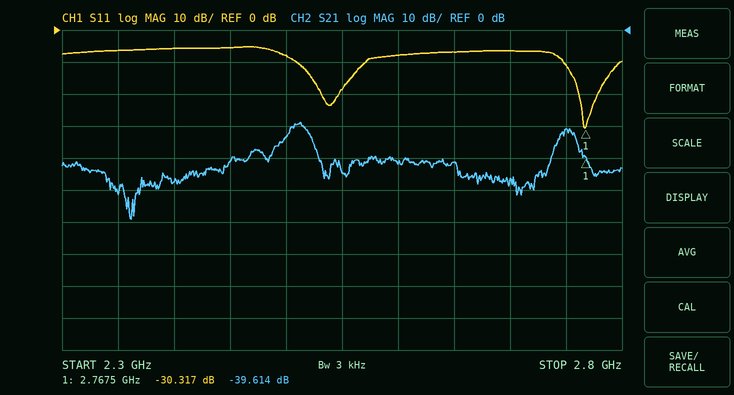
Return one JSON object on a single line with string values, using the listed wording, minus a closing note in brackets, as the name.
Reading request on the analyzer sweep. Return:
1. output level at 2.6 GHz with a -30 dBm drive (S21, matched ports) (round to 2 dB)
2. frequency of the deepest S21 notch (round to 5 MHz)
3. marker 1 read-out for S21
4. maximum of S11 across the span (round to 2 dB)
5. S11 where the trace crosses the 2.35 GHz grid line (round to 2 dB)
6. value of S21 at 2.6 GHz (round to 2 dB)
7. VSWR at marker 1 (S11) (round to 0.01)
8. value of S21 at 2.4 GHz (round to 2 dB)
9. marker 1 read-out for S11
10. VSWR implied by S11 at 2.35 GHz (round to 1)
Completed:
{"output level at 2.6 GHz with a -30 dBm drive (S21, matched ports)": "-72 dBm", "frequency of the deepest S21 notch": "2.360 GHz", "marker 1 read-out for S21": "-39.614 dB", "maximum of S11 across the span": "-6 dB", "S11 where the trace crosses the 2.35 GHz grid line": "-6 dB", "value of S21 at 2.6 GHz": "-42 dB", "VSWR at marker 1 (S11)": "1.06", "value of S21 at 2.4 GHz": "-48 dB", "marker 1 read-out for S11": "-30.317 dB", "VSWR implied by S11 at 2.35 GHz": "3"}
